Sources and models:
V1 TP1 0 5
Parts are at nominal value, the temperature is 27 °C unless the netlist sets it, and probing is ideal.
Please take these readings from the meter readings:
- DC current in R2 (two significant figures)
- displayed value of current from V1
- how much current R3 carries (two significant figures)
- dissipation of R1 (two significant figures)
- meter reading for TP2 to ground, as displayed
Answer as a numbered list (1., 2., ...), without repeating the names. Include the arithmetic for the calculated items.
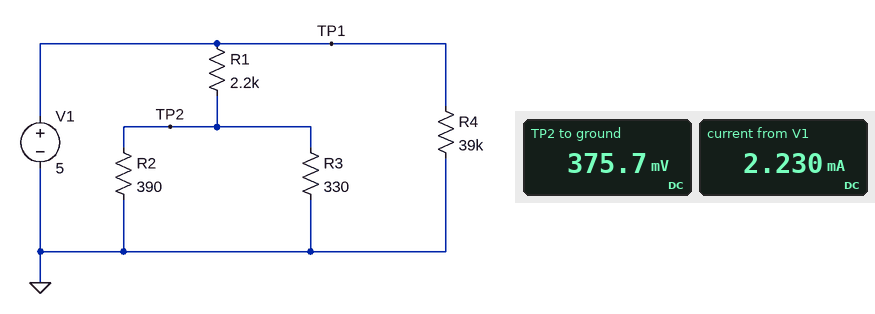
1. (375.7 mV) / 390 Ω = 960 µA
2. 2.230 mA
3. (375.7 mV) / 330 Ω = 1.1 mA
4. (5 V - 375.7 mV)^2 / 2.2 kΩ = 9.7 mW
5. 375.7 mV
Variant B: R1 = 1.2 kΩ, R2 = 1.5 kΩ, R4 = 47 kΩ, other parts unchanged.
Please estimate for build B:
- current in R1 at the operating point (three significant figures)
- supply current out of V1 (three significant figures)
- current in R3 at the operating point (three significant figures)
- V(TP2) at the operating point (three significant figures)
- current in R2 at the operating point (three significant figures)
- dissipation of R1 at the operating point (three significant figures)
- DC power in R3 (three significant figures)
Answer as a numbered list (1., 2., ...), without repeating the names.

1. 3.40 mA
2. 3.51 mA
3. 2.79 mA
4. 920 mV
5. 613 µA
6. 13.9 mW
7. 2.56 mW
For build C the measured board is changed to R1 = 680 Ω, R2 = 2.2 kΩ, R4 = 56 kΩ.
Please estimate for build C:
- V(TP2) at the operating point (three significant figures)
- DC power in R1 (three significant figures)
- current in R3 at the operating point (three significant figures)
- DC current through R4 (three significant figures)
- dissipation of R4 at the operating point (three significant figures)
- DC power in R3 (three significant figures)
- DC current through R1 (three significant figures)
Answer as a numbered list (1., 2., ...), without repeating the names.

1. 1.48 V
2. 18.2 mW
3. 4.50 mA
4. 89.3 µA
5. 446 µW
6. 6.67 mW
7. 5.17 mA
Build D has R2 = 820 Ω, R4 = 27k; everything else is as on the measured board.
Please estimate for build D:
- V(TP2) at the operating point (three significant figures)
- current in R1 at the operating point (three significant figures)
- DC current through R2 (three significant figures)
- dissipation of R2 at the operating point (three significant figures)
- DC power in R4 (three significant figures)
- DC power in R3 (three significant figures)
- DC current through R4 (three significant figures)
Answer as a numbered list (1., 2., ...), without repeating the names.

1. 483 mV
2. 2.05 mA
3. 589 µA
4. 285 µW
5. 926 µW
6. 707 µW
7. 185 µA
